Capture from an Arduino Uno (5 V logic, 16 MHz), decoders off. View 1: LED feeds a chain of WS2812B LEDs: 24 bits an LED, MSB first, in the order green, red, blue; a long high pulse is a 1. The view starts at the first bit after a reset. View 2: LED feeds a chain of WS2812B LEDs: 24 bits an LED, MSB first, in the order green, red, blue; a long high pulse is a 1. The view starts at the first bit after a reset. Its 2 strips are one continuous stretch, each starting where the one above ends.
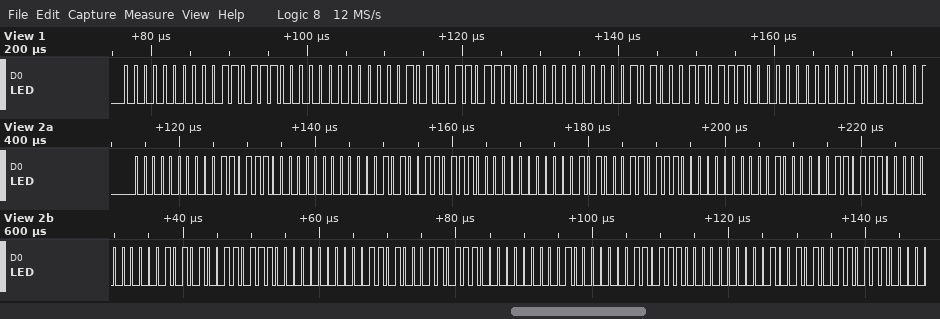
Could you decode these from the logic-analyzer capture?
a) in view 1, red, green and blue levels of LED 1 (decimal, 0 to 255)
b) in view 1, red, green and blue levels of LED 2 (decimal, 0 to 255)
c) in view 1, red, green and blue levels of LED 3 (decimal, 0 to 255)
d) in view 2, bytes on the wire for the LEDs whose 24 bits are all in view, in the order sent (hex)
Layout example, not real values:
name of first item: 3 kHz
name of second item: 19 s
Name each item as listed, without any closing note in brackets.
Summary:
in view 1, red, green and blue levels of LED 1: 55, 0, 0
in view 1, red, green and blue levels of LED 2: 55, 5, 0
in view 1, red, green and blue levels of LED 3: 55, 10, 0
in view 2, bytes on the wire for the LEDs whose 24 bits are all in view, in the order sent: 00 37 00 05 37 00 0A 37 00 10 37 00 15 37 00 1A 37 00 20 37 00
